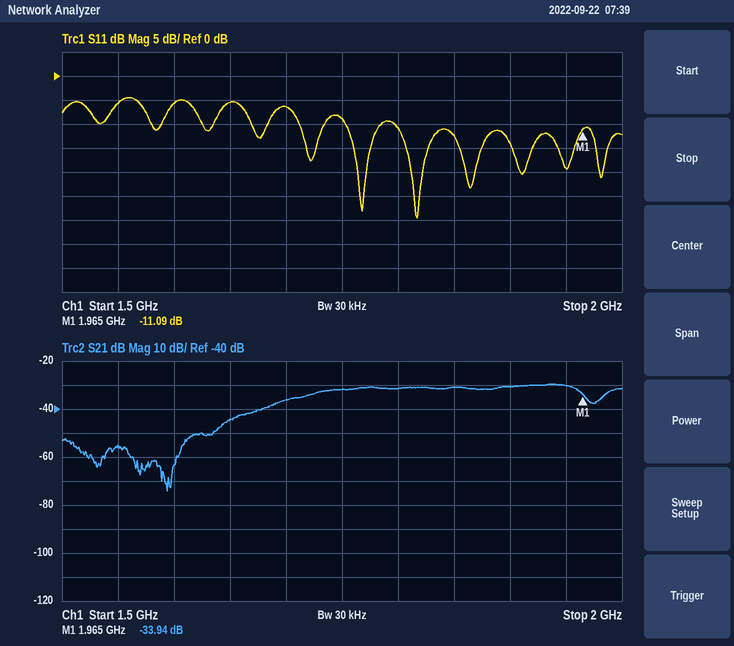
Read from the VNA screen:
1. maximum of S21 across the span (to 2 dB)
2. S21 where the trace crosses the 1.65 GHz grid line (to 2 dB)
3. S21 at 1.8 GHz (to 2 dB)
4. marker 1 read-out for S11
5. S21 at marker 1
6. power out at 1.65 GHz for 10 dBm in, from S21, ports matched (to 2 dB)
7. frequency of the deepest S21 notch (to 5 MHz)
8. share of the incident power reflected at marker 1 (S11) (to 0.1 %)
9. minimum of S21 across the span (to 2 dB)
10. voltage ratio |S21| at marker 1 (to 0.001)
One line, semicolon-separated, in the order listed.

-30 dB; -44 dB; -32 dB; -11.09 dB; -33.94 dB; -34 dBm; 1.595 GHz; 7.8 %; -74 dB; 0.020
